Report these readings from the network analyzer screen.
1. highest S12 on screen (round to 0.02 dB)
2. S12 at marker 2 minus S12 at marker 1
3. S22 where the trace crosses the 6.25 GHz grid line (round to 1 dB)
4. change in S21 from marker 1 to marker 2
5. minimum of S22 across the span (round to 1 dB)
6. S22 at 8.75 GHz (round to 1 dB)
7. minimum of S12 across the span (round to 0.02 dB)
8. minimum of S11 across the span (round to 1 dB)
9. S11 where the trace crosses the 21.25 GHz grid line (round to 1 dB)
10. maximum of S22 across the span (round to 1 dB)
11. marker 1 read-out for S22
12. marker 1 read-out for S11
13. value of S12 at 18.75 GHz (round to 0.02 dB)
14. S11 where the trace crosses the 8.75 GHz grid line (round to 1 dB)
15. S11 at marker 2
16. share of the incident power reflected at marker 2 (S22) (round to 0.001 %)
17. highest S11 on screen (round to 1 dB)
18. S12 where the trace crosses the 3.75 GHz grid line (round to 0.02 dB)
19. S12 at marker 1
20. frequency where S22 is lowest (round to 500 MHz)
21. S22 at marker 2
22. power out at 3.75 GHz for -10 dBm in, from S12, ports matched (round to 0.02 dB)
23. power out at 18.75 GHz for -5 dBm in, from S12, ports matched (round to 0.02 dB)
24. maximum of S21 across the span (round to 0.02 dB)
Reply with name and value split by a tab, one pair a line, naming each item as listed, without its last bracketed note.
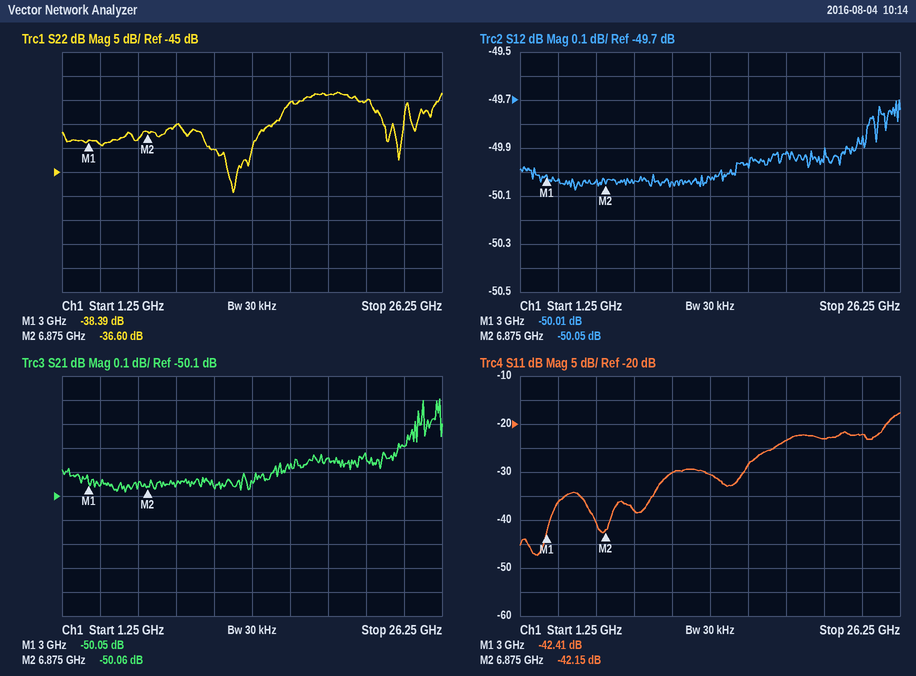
highest S12 on screen	-49.70 dB
S12 at marker 2 minus S12 at marker 1	-0.04 dB
S22 where the trace crosses the 6.25 GHz grid line	-38 dB
change in S21 from marker 1 to marker 2	-0.01 dB
minimum of S22 across the span	-49 dB
S22 at 8.75 GHz	-35 dB
minimum of S12 across the span	-50.08 dB
minimum of S11 across the span	-47 dB
S11 where the trace crosses the 21.25 GHz grid line	-23 dB
maximum of S22 across the span	-28 dB
marker 1 read-out for S22	-38.39 dB
marker 1 read-out for S11	-42.41 dB
value of S12 at 18.75 GHz	-49.92 dB
S11 where the trace crosses the 8.75 GHz grid line	-38 dB
S11 at marker 2	-42.15 dB
share of the incident power reflected at marker 2 (S22)	0.022 %
highest S11 on screen	-18 dB
S12 where the trace crosses the 3.75 GHz grid line	-50.04 dB
S12 at marker 1	-50.01 dB
frequency where S22 is lowest	12.5 GHz
S22 at marker 2	-36.60 dB
power out at 3.75 GHz for -10 dBm in, from S12, ports matched	-60.04 dBm
power out at 18.75 GHz for -5 dBm in, from S12, ports matched	-54.92 dBm
maximum of S21 across the span	-49.70 dB
